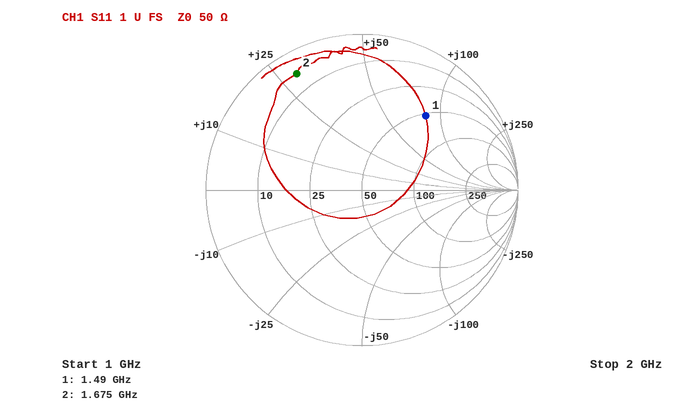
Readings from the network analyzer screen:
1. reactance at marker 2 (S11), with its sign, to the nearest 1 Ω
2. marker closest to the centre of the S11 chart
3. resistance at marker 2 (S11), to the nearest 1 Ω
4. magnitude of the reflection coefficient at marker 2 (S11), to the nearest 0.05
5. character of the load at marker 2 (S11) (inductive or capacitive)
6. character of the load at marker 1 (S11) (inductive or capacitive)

+29 Ω
marker 1
5 Ω
0.85
inductive
inductive
